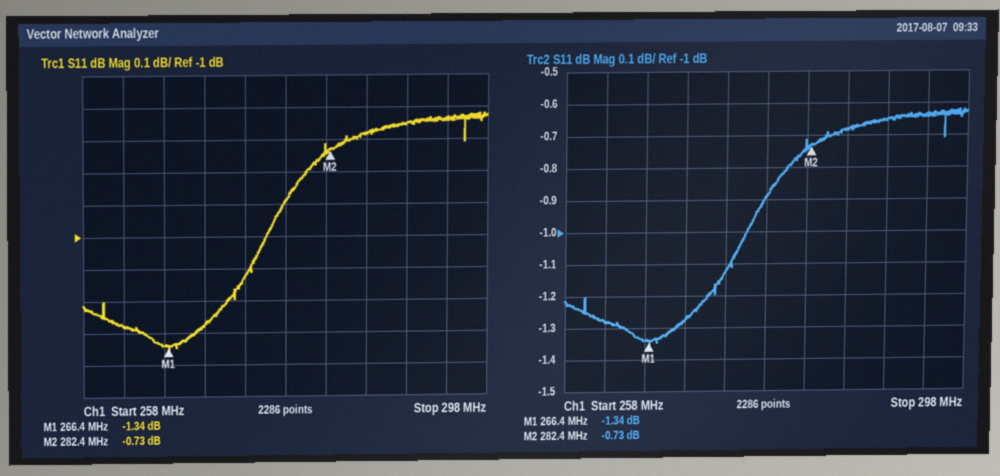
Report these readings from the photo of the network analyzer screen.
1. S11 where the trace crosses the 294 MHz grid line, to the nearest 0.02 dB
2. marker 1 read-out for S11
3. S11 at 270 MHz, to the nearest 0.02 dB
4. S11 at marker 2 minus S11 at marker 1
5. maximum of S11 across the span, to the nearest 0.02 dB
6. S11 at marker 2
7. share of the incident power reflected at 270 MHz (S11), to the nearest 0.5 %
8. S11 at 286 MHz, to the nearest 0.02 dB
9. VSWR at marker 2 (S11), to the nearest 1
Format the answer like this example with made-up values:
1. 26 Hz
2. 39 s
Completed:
1. -0.64 dB
2. -1.34 dB
3. -1.28 dB
4. 0.61 dB
5. -0.62 dB
6. -0.73 dB
7. 74.5 %
8. -0.68 dB
9. 24
